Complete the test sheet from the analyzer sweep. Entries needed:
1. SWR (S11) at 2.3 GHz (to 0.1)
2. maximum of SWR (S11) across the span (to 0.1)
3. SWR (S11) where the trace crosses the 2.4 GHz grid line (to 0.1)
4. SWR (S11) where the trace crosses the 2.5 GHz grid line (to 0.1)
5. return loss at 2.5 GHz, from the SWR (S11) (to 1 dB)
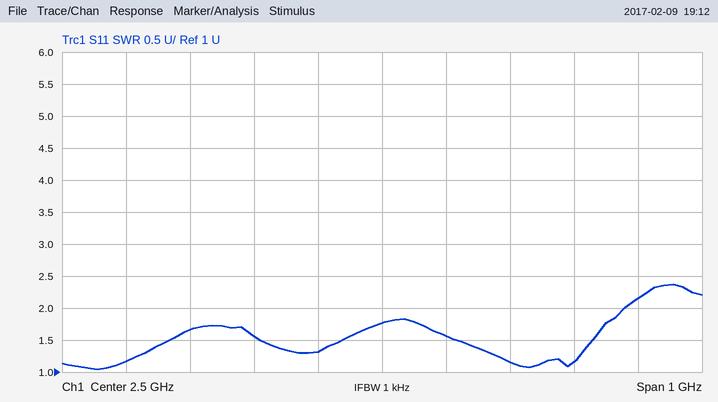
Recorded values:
1.6
2.4
1.3
1.8
11 dB
